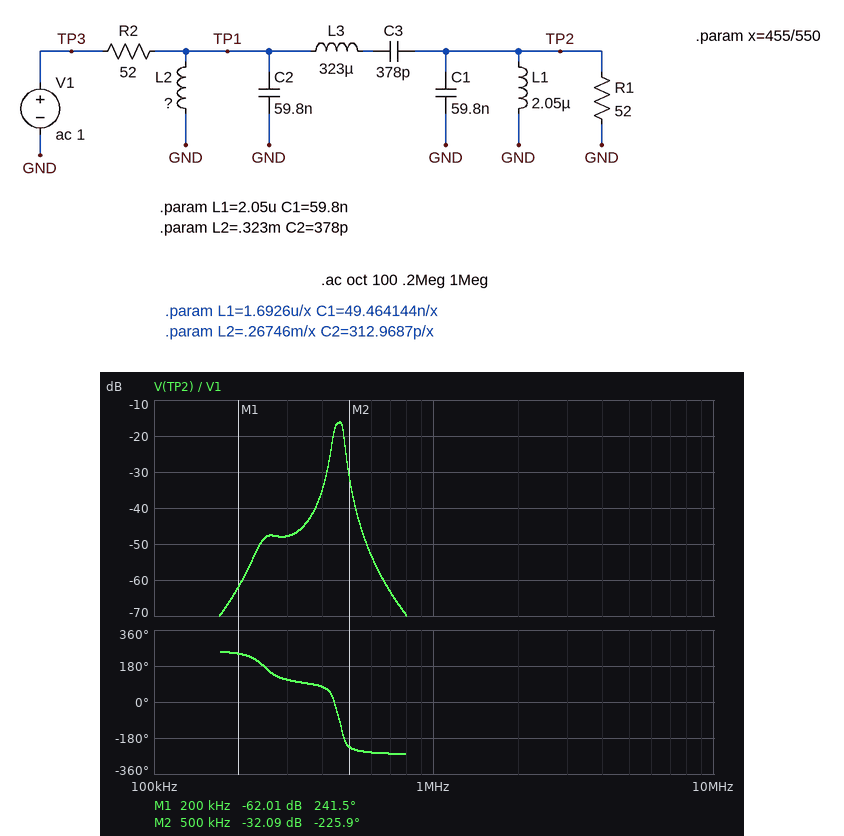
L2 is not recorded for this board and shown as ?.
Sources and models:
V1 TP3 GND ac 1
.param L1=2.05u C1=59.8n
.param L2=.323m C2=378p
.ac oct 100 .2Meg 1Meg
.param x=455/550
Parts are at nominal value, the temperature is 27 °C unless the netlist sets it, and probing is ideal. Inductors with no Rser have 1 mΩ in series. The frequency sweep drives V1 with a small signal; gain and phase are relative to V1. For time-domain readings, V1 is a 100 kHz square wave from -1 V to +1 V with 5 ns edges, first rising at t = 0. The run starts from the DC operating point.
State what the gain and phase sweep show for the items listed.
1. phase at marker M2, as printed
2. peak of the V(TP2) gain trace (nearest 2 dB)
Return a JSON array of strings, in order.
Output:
["-225.9 deg", "-16 dB"]
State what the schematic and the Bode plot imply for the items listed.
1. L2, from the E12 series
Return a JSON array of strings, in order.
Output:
["6.8 µH"]
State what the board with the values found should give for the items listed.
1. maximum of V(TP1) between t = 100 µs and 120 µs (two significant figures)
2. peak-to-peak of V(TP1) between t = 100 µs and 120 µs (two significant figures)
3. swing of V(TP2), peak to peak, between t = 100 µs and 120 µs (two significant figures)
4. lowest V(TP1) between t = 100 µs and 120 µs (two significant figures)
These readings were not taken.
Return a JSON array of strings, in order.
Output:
["300 mV", "590 mV", "16 mV", "-300 mV"]
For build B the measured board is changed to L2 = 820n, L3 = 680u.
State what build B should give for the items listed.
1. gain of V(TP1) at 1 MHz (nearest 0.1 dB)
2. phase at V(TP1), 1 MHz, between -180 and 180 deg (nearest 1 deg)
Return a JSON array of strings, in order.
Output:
["-19.5 dB", "-84 deg"]
